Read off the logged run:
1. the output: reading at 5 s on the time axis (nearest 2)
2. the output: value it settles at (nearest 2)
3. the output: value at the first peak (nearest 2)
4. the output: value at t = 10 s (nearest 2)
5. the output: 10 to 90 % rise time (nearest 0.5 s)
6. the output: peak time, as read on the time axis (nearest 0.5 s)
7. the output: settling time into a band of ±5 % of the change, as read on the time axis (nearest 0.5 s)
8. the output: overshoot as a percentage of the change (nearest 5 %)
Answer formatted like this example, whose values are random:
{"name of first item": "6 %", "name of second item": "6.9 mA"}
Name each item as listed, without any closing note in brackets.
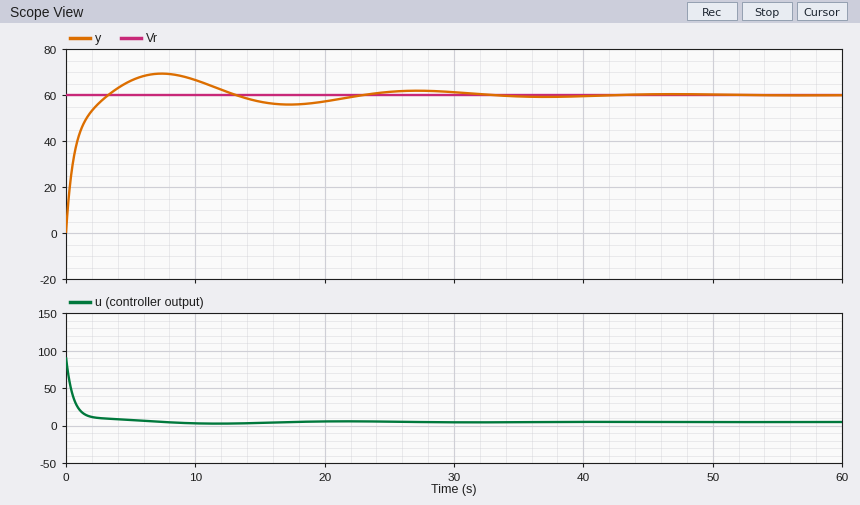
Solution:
{"the output: reading at 5 s on the time axis": "66", "the output: value it settles at": "60", "the output: value at the first peak": "70", "the output: value at t = 10 s": "66", "the output: 10 to 90 % rise time": "2.0 s", "the output: peak time, as read on the time axis": "7.5 s", "the output: settling time into a band of ±5 % of the change, as read on the time axis": "20.0 s", "the output: overshoot as a percentage of the change": "15 %"}
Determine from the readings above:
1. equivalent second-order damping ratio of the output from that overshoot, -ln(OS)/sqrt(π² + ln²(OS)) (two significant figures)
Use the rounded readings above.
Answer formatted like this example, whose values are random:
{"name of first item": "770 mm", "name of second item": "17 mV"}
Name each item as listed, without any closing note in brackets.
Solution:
{"equivalent second-order damping ratio of the output from that overshoot, -ln(OS)/sqrt(π² + ln²(OS))": "0.52"}
